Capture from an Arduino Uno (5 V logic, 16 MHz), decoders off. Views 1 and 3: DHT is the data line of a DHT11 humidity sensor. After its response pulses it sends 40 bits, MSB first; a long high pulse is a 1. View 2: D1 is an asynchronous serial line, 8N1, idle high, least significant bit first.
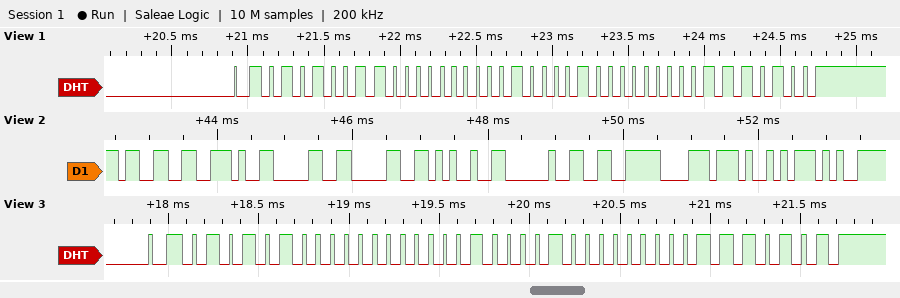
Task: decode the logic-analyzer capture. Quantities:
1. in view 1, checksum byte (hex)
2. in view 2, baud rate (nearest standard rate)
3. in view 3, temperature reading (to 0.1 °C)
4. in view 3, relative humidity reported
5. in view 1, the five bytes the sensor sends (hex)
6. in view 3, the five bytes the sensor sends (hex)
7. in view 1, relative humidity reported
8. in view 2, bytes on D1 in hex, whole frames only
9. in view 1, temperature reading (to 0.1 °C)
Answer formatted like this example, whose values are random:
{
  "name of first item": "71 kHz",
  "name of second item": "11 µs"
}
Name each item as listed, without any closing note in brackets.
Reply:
{
  "in view 1, checksum byte": "0x74",
  "in view 2, baud rate": "9600 baud",
  "in view 3, temperature reading": "33.0 °C",
  "in view 3, relative humidity reported": "84 %",
  "in view 1, the five bytes the sensor sends": "53 00 21 00 74",
  "in view 3, the five bytes the sensor sends": "54 00 21 00 75",
  "in view 1, relative humidity reported": "83 %",
  "in view 2, bytes on D1 in hex, whole frames only": "0x33 0x2E 0x30 0x30 0x25 0x20 0xE6 0xB8 0xA9 0xE5",
  "in view 1, temperature reading": "33.0 °C"
}
